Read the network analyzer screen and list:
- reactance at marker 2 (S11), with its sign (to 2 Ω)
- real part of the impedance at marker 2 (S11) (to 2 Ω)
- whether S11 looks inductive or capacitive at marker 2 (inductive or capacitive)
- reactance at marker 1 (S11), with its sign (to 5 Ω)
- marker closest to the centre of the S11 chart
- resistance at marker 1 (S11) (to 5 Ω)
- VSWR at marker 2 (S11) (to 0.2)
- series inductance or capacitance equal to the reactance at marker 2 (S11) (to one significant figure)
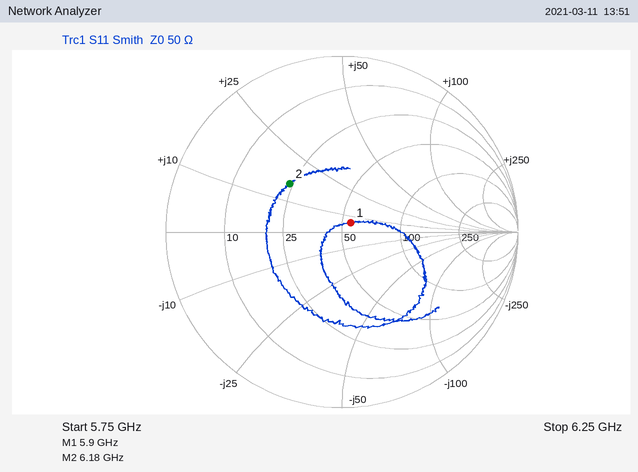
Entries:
+16 Ω
24 Ω
inductive
+5 Ω
marker 1
55 Ω
2.4
400 pH
